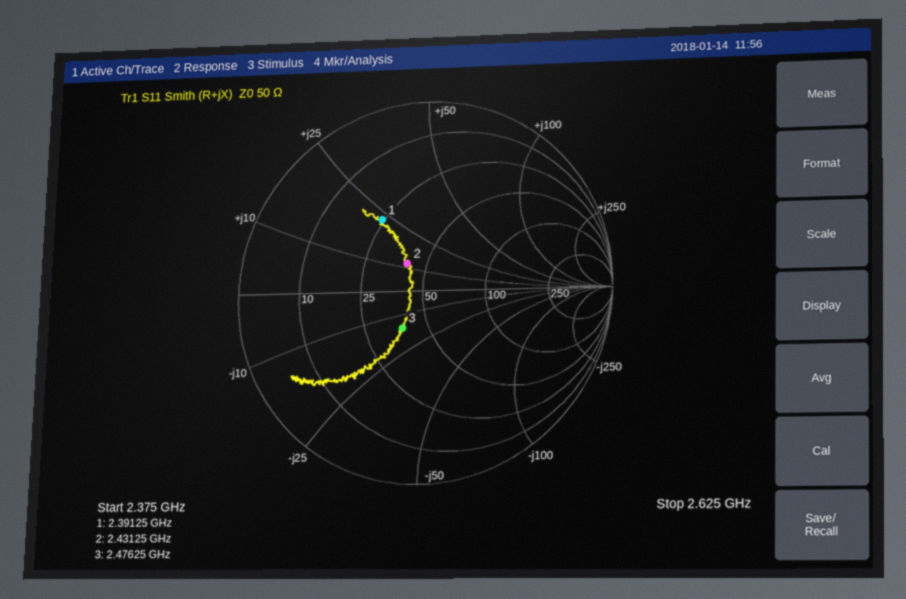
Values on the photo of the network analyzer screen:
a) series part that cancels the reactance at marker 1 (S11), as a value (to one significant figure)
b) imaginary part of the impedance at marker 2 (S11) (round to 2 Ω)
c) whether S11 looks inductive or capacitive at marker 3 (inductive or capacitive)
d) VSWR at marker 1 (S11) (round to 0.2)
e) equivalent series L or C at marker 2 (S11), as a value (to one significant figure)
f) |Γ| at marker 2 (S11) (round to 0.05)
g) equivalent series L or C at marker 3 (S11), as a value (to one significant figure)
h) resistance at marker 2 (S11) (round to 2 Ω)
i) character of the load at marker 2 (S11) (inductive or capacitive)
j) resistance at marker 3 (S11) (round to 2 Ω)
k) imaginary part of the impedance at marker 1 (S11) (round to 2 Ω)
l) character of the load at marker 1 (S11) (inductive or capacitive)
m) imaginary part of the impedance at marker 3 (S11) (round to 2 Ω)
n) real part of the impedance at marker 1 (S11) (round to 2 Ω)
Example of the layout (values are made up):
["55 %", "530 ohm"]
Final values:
["3 pF", "+12 Ω", "capacitive", "2.6", "800 pH", "0.15", "4 pF", "40 Ω", "inductive", "38 Ω", "+22 Ω", "inductive", "-16 Ω", "24 Ω"]
